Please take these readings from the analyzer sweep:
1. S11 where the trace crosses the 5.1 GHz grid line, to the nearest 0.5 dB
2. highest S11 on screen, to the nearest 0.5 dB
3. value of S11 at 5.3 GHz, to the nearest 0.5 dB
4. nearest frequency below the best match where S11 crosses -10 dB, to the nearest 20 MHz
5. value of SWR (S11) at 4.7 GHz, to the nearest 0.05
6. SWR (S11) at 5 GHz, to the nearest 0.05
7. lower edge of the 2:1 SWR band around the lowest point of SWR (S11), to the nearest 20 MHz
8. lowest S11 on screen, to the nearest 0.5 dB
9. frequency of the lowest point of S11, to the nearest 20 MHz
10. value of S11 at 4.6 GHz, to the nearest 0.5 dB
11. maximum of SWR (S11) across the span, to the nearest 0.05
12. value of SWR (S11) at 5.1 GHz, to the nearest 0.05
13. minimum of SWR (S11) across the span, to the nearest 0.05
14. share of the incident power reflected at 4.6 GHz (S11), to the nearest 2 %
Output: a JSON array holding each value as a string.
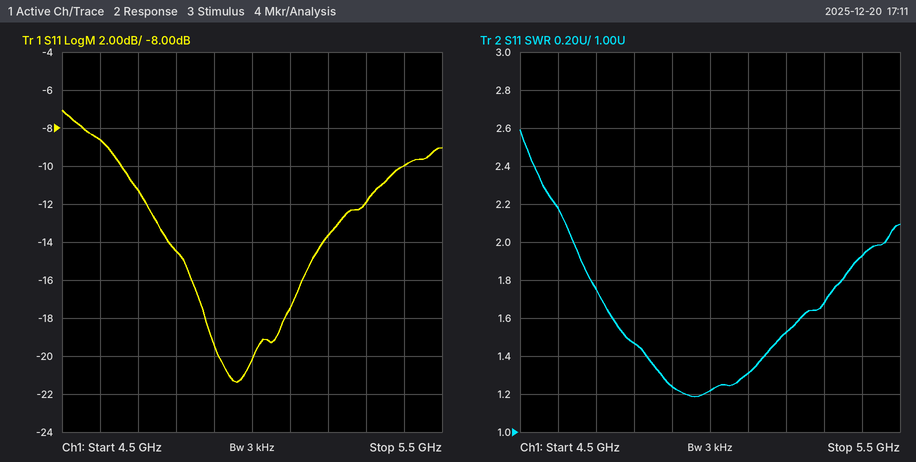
["-17.5 dB", "-7.0 dB", "-12.0 dB", "4.66 GHz", "1.75", "1.20", "4.64 GHz", "-21.5 dB", "4.96 GHz", "-8.5 dB", "2.60", "1.30", "1.20", "14 %"]
